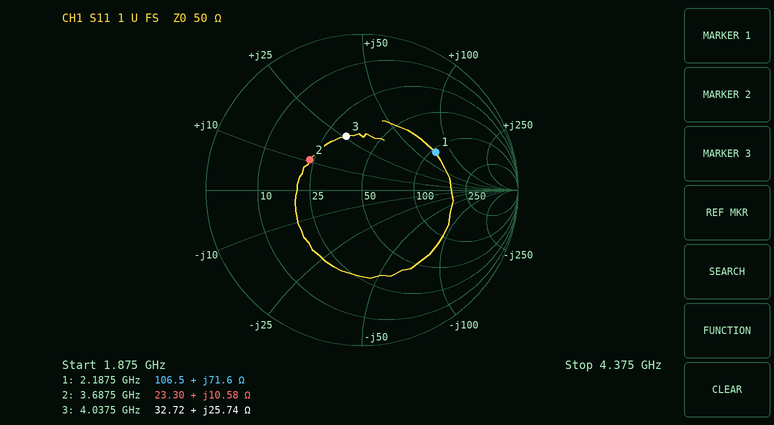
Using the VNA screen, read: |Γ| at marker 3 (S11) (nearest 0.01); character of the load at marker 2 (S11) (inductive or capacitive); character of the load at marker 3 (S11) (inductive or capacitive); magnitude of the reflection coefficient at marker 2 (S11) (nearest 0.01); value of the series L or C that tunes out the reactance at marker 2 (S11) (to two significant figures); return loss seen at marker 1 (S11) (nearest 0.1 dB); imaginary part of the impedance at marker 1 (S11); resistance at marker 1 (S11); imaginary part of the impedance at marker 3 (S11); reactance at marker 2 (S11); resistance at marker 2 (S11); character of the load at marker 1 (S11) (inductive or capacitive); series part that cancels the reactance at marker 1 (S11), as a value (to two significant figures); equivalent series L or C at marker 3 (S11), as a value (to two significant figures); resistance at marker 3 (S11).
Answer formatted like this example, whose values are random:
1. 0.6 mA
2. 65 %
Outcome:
1. 0.36
2. inductive
3. inductive
4. 0.39
5. 4.1 pF
6. 5.5 dB
7. +71.6 Ω
8. 106.5 Ω
9. +25.74 Ω
10. +10.58 Ω
11. 23.30 Ω
12. inductive
13. 1.0 pF
14. 1.0 nH
15. 32.72 Ω
